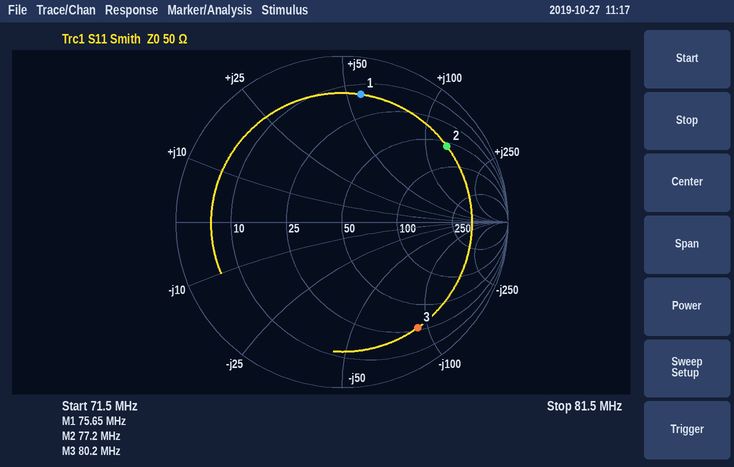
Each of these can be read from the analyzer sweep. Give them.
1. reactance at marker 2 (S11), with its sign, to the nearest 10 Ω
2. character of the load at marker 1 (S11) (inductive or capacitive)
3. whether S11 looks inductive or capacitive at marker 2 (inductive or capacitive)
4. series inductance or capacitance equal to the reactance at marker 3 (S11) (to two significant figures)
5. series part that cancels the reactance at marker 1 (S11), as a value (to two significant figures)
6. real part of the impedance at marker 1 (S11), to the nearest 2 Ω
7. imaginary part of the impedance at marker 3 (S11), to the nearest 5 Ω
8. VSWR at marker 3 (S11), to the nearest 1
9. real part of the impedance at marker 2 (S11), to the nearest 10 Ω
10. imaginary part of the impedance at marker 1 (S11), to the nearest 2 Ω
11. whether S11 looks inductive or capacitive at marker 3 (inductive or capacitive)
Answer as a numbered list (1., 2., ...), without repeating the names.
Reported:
1. +130 Ω
2. inductive
3. inductive
4. 22 pF
5. 38 pF
6. 14 Ω
7. -90 Ω
8. 8
9. 60 Ω
10. +56 Ω
11. capacitive
